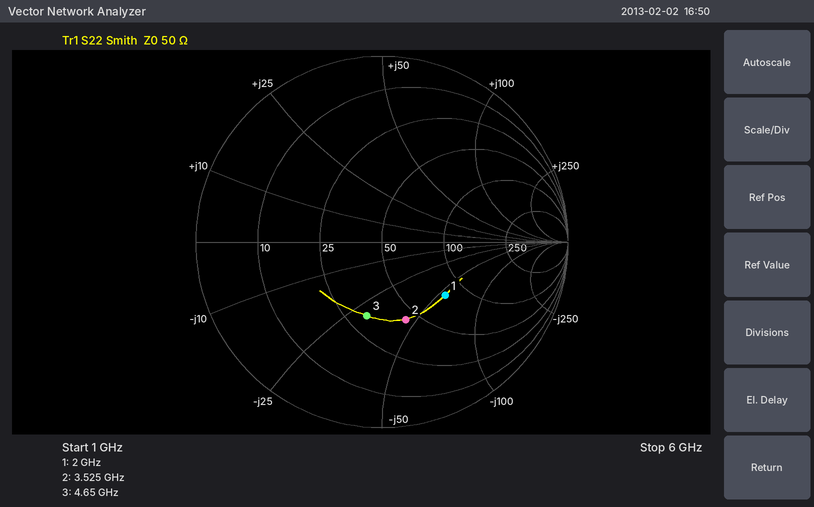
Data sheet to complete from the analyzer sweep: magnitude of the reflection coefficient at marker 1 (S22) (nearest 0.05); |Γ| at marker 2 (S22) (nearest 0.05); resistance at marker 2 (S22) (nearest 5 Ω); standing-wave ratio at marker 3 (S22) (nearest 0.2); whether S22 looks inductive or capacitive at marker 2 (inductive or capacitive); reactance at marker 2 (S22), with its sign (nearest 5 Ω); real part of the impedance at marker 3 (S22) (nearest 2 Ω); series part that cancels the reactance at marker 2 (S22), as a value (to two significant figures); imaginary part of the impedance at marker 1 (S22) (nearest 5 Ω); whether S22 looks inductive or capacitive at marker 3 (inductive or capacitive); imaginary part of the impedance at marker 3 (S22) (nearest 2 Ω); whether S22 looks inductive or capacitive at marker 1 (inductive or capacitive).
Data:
0.45
0.45
45 Ω
2.4
capacitive
-45 Ω
32 Ω
2.0 nH
-55 Ω
capacitive
-30 Ω
capacitive
